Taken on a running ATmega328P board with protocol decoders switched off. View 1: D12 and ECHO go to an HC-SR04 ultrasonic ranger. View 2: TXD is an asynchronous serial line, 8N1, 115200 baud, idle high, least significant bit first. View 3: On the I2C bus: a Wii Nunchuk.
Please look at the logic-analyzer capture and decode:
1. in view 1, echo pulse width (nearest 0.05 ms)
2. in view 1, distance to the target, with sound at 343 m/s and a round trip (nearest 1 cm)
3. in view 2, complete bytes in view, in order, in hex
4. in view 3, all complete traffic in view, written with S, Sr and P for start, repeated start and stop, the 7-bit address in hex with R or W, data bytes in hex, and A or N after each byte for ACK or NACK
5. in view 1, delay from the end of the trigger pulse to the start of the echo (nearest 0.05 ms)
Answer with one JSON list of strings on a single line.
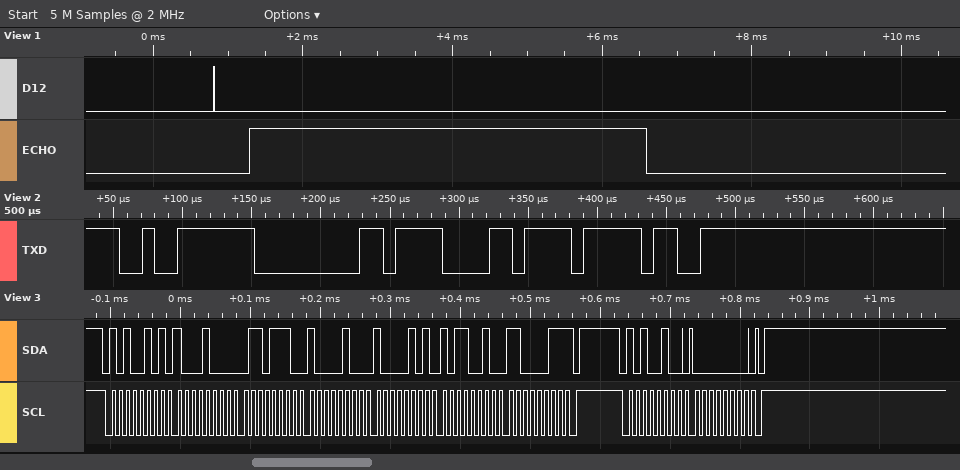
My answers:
["5.30 ms", "91 cm", "0xF2 0x00 0x0F 0xEF 0xF3", "S 52R A 88 A 6E A 84 A 85 A B2 A C3 N P S 52W A 00 A P", "0.45 ms"]
